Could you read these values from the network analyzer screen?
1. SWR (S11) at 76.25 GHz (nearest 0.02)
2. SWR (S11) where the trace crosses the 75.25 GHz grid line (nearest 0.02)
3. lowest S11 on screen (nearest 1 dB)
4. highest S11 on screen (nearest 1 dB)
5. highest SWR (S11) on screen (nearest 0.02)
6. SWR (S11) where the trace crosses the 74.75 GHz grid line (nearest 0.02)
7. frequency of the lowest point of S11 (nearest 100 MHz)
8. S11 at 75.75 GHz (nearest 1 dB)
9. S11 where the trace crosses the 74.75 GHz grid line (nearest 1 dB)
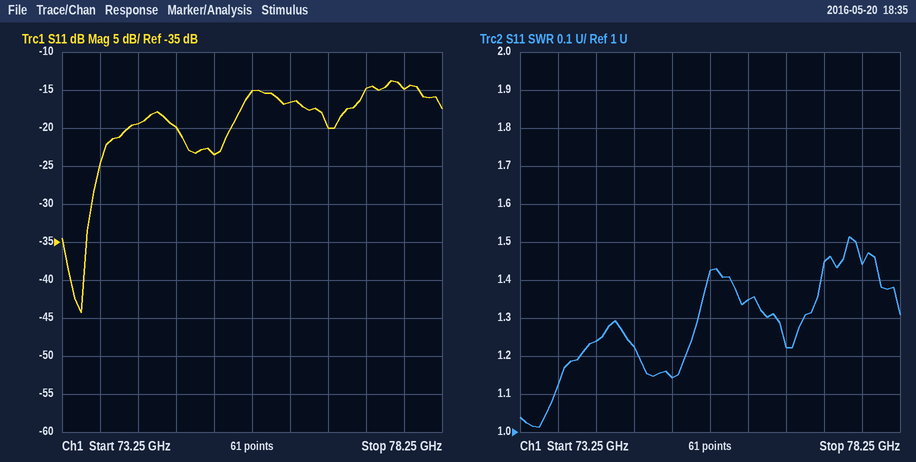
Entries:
1.34
1.14
-44 dB
-14 dB
1.52
1.22
73.5 GHz
-15 dB
-20 dB
